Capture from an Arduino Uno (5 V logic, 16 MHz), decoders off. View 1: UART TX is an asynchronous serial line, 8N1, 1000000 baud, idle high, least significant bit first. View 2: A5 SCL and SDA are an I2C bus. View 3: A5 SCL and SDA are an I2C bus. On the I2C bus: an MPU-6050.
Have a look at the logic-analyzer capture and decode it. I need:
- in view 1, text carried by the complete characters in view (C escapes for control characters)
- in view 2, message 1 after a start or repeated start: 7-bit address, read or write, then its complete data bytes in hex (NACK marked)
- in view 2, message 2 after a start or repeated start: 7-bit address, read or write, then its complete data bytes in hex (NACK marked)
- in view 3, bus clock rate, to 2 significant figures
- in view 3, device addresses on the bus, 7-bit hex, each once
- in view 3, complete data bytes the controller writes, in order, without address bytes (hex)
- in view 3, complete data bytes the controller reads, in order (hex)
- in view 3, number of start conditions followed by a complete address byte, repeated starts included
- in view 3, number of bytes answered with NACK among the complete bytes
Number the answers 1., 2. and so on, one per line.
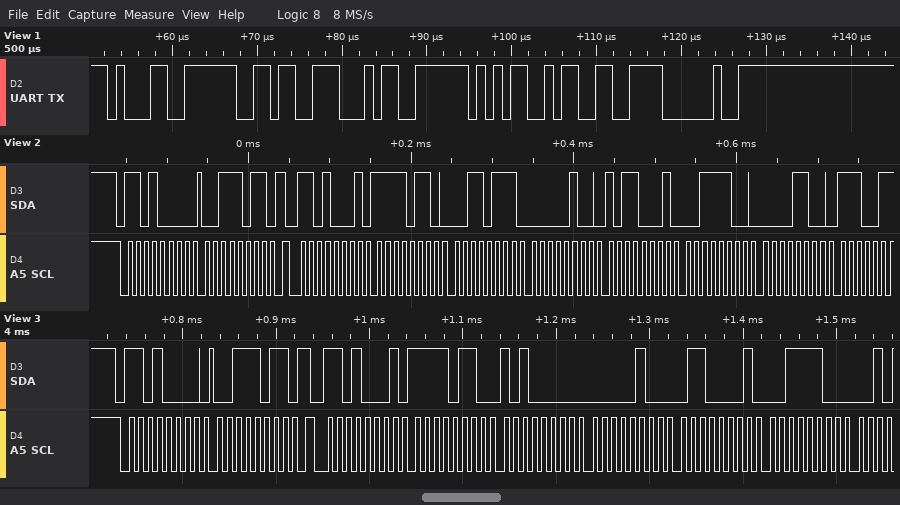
1. "16453 "
2. 0x68 write: 3B
3. 0x68 read: F6 37 04 B1 3C 0C
4. 100 kHz
5. 0x68
6. 3B
7. F6 A0 04 61 3C
8. 2
9. 0
